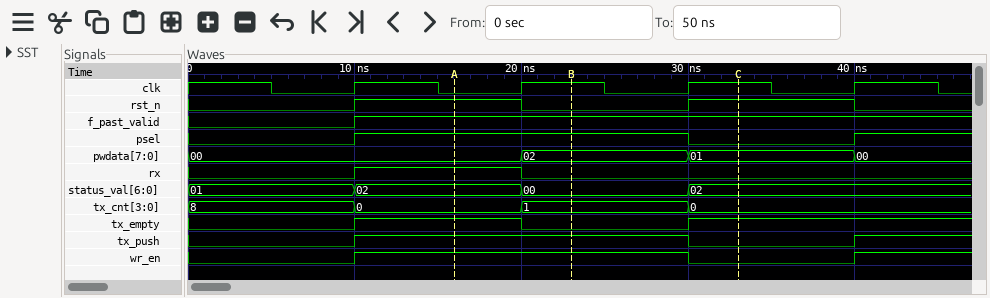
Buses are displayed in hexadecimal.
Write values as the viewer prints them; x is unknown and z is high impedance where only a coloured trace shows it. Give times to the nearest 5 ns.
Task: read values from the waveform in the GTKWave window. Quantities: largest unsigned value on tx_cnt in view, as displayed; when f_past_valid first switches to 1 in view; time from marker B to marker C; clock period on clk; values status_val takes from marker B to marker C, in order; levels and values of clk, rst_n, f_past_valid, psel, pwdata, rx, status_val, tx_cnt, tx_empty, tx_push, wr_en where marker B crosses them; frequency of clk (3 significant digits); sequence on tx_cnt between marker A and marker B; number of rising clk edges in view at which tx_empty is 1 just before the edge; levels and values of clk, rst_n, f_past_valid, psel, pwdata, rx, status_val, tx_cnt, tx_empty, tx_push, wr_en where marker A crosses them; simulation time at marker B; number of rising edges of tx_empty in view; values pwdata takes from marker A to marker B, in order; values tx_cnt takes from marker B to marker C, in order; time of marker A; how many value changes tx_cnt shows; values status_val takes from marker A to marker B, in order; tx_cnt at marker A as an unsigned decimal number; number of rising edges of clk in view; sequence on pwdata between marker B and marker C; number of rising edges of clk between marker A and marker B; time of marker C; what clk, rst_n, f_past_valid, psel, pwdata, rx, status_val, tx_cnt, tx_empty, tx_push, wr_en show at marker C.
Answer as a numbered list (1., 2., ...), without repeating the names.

1. 8
2. 10 ns
3. 10 ns
4. 10 ns
5. 00, 02
6. clk=1, rst_n=0, f_past_valid=1, psel=1, pwdata=02, rx=0, status_val=00, tx_cnt=1, tx_empty=0, tx_push=1, wr_en=1
7. 100 MHz
8. 0, 1
9. 2
10. clk=0, rst_n=1, f_past_valid=1, psel=1, pwdata=00, rx=1, status_val=02, tx_cnt=0, tx_empty=1, tx_push=1, wr_en=1
11. 25 ns
12. 2
13. 00, 02
14. 1, 0
15. 15 ns
16. 3
17. 02, 00
18. 0
19. 4
20. 02, 01
21. 1
22. 35 ns
23. clk=1, rst_n=1, f_past_valid=1, psel=0, pwdata=01, rx=0, status_val=02, tx_cnt=0, tx_empty=1, tx_push=0, wr_en=0
